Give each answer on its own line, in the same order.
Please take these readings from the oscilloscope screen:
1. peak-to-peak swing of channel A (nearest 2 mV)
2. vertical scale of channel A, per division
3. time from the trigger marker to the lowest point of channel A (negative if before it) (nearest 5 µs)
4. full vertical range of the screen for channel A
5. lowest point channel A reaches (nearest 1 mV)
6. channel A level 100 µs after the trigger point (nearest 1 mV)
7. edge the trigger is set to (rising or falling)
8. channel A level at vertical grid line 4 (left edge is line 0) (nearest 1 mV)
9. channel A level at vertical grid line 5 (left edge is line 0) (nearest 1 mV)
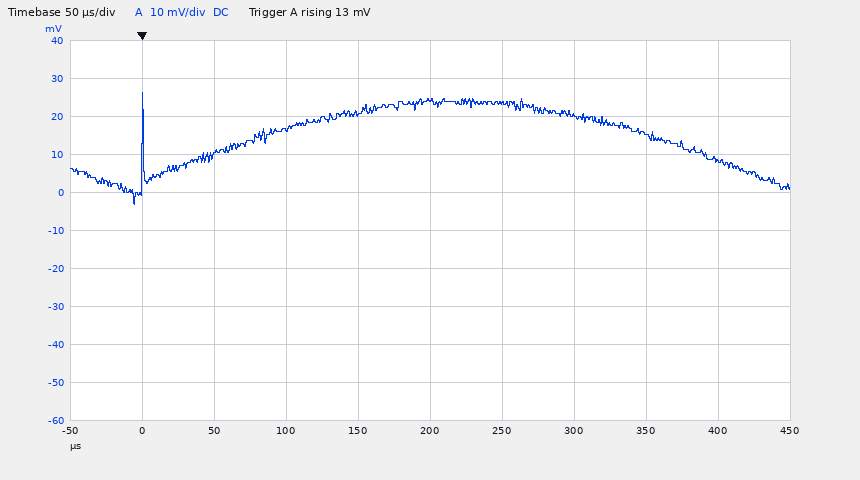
30 mV
10 mV
-5 µs
100 mV
-3 mV
17 mV
rising
21 mV
24 mV
